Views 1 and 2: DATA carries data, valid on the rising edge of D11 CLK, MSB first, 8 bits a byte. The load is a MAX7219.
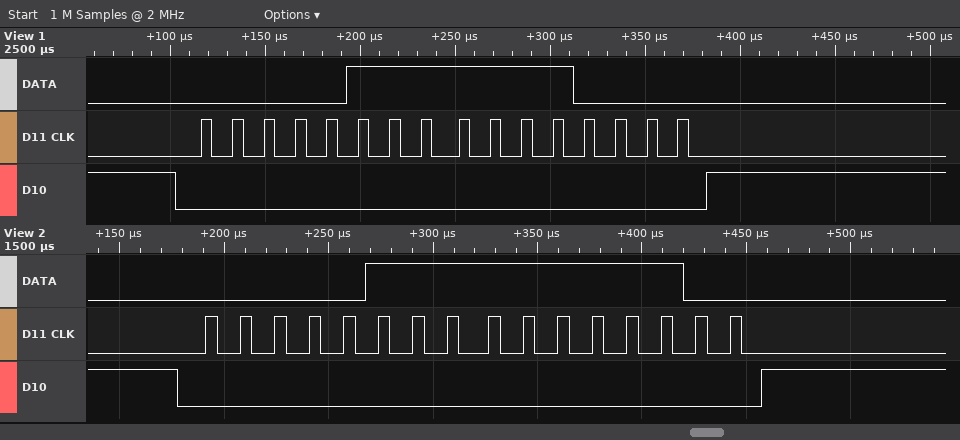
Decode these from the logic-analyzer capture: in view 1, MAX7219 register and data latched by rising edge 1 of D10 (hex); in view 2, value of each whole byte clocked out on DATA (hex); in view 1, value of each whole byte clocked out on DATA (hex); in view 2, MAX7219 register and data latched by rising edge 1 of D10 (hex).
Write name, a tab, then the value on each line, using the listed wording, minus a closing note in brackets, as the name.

in view 1, MAX7219 register and data latched by rising edge 1 of D10	register 0x7, data 0xF0
in view 2, value of each whole byte clocked out on DATA	07 FC
in view 1, value of each whole byte clocked out on DATA	07 F0
in view 2, MAX7219 register and data latched by rising edge 1 of D10	register 0x7, data 0xFC
